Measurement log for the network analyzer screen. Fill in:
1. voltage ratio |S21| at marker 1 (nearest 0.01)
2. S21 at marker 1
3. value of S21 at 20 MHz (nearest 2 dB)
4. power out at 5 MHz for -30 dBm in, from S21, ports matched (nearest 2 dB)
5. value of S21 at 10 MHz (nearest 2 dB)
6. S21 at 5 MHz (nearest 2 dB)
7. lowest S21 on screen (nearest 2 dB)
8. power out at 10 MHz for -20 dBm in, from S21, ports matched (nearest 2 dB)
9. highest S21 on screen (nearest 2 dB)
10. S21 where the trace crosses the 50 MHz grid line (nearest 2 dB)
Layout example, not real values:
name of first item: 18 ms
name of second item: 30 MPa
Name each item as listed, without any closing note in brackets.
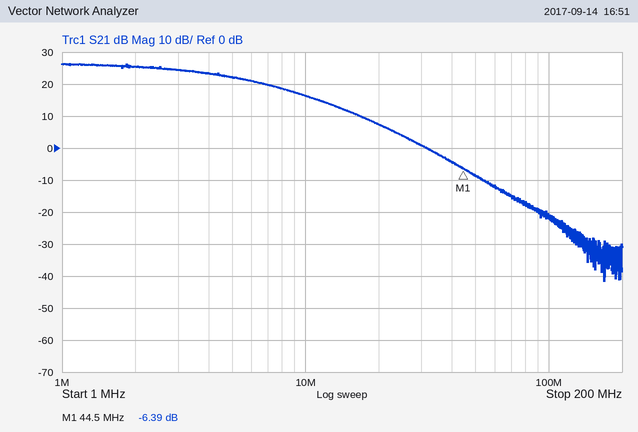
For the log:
voltage ratio |S21| at marker 1: 0.48
S21 at marker 1: -6.39 dB
value of S21 at 20 MHz: 8 dB
power out at 5 MHz for -30 dBm in, from S21, ports matched: -8 dBm
value of S21 at 10 MHz: 16 dB
S21 at 5 MHz: 22 dB
lowest S21 on screen: -42 dB
power out at 10 MHz for -20 dBm in, from S21, ports matched: -4 dBm
highest S21 on screen: 26 dB
S21 where the trace crosses the 50 MHz grid line: -8 dB
